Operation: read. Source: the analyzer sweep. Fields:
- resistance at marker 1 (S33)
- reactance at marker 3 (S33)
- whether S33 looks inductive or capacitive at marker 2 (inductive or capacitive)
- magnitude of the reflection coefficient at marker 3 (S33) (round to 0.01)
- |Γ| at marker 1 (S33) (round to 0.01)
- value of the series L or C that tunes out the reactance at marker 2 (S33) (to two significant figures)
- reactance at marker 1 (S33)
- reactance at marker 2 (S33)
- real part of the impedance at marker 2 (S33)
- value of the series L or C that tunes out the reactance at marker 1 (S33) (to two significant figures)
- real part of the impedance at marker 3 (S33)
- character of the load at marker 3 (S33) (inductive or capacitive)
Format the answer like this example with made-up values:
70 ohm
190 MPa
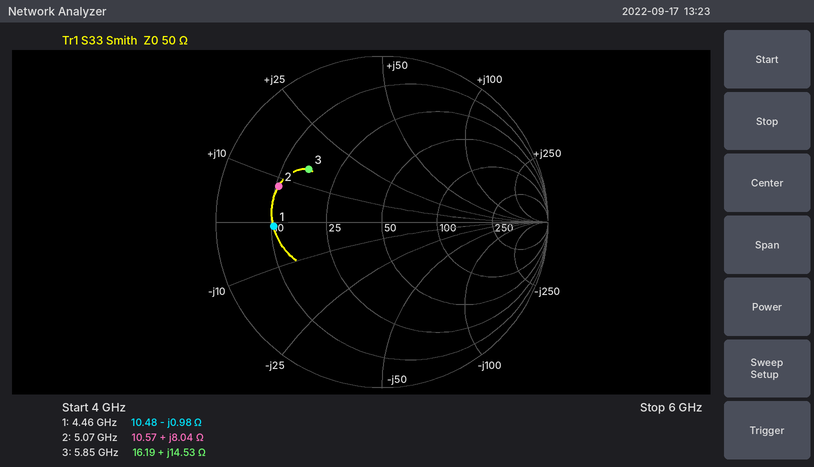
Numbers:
10.48 Ω
+14.53 Ω
inductive
0.54
0.65
3.9 pF
-0.98 Ω
+8.04 Ω
10.57 Ω
35 pH
16.19 Ω
inductive
